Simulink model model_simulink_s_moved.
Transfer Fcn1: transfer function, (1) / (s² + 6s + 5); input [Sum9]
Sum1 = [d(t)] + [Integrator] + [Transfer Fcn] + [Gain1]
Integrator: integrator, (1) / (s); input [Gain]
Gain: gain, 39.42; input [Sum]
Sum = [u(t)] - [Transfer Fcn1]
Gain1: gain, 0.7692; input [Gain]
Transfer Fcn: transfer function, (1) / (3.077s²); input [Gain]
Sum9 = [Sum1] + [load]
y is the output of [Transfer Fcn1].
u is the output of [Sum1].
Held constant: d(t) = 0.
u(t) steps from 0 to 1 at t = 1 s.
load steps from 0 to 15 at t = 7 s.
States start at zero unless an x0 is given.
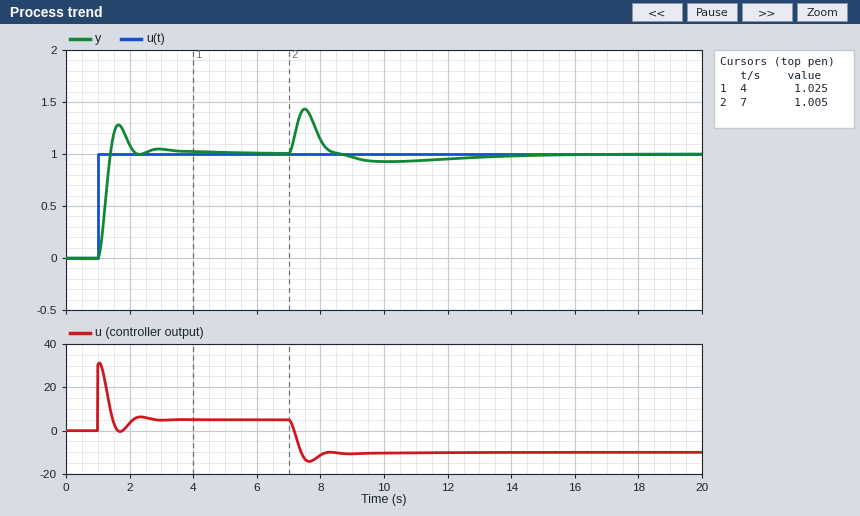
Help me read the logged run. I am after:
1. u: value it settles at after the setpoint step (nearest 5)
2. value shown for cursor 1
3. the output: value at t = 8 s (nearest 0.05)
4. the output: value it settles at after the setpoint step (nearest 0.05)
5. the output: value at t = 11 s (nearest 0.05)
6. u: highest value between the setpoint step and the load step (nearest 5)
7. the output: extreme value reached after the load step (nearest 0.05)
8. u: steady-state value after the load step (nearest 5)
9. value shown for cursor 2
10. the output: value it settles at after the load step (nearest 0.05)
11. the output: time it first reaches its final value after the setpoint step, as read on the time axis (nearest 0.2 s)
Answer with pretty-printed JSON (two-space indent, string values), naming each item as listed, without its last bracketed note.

{
  "u: value it settles at after the setpoint step": "5",
  "value shown for cursor 1": "1.025",
  "the output: value at t = 8 s": "1.15",
  "the output: value it settles at after the setpoint step": "1.00",
  "the output: value at t = 11 s": "0.95",
  "u: highest value between the setpoint step and the load step": "30",
  "the output: extreme value reached after the load step": "1.45",
  "u: steady-state value after the load step": "-10",
  "value shown for cursor 2": "1.005",
  "the output: value it settles at after the load step": "1.00",
  "the output: time it first reaches its final value after the setpoint step, as read on the time axis": "1.4 s"
}
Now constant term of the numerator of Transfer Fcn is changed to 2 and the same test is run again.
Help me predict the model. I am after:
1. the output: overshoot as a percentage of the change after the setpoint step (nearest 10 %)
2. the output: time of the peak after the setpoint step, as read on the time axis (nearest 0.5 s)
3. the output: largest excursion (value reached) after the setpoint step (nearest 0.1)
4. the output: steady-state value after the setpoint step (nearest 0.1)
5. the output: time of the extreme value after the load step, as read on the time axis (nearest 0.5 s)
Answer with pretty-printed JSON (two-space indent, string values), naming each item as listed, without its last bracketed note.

{
  "the output: overshoot as a percentage of the change after the setpoint step": "30 %",
  "the output: time of the peak after the setpoint step, as read on the time axis": "1.5 s",
  "the output: largest excursion (value reached) after the setpoint step": "1.3",
  "the output: steady-state value after the setpoint step": "1.0",
  "the output: time of the extreme value after the load step, as read on the time axis": "7.5 s"
}
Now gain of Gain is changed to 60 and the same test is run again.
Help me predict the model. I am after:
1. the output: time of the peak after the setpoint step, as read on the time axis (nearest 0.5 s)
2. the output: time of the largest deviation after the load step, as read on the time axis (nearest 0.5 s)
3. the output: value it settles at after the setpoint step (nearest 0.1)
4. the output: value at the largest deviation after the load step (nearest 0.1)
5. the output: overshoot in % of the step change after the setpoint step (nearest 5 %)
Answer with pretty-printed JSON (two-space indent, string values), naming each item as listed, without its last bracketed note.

{
  "the output: time of the peak after the setpoint step, as read on the time axis": "1.5 s",
  "the output: time of the largest deviation after the load step, as read on the time axis": "7.5 s",
  "the output: value it settles at after the setpoint step": "1.0",
  "the output: value at the largest deviation after the load step": "1.3",
  "the output: overshoot in % of the step change after the setpoint step": "35 %"
}
